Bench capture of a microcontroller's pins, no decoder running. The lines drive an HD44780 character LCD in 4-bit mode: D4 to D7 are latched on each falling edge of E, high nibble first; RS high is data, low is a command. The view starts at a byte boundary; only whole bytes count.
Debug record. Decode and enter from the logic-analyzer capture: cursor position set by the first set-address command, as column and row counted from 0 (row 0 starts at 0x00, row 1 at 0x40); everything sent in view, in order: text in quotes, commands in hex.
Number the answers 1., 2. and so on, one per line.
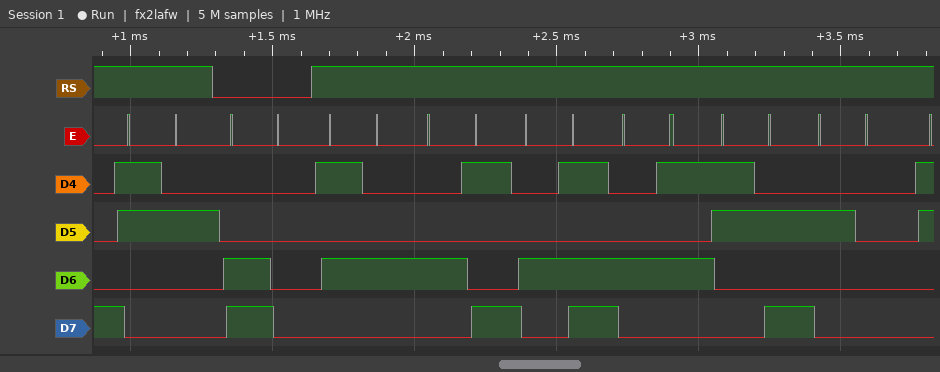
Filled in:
1. column 0, row 1
2. "2" 0xC0 "TIME: "
